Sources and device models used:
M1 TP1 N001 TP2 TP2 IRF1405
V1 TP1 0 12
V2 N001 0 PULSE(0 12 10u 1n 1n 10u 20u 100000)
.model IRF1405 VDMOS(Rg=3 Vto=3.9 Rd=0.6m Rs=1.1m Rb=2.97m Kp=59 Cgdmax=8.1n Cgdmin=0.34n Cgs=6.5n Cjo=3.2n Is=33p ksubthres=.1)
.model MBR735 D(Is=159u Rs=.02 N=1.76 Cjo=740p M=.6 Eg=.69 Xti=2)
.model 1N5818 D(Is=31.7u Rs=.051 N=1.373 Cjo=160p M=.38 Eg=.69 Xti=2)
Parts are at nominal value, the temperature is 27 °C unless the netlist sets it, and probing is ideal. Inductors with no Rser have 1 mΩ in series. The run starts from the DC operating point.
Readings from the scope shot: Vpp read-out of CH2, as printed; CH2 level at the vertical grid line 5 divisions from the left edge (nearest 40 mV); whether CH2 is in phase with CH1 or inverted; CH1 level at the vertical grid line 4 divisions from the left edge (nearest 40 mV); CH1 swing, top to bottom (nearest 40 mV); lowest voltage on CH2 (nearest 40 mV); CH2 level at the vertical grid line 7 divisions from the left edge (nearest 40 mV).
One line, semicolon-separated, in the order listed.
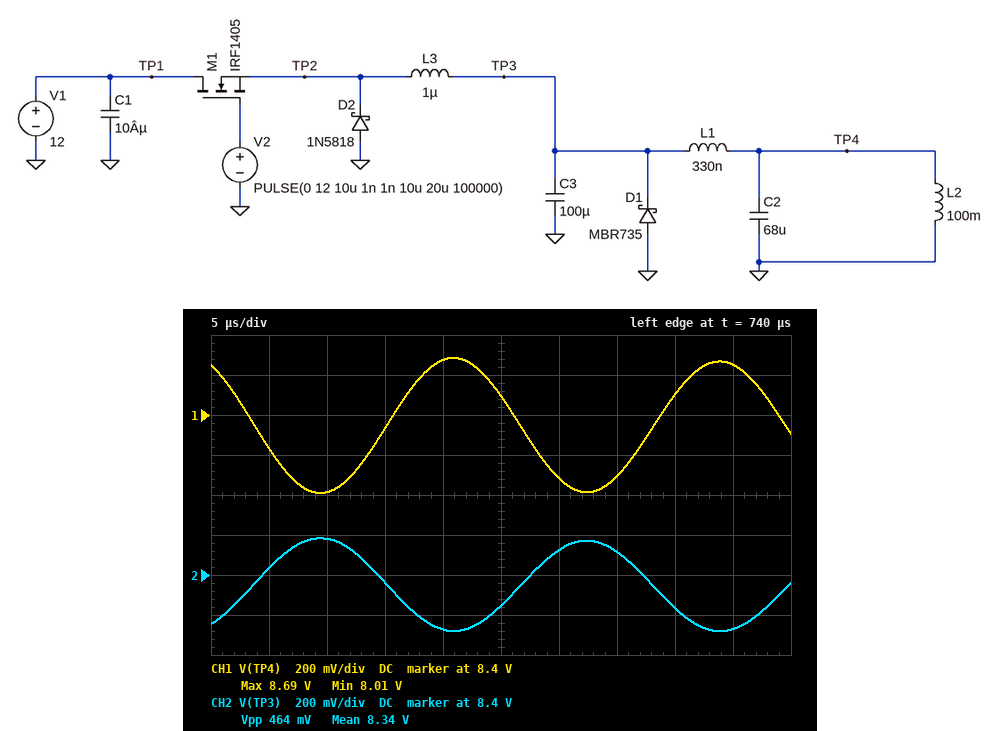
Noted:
464 mV; 8.24 V; inverted; 8.68 V; 680 mV; 8.12 V; 8.52 V
